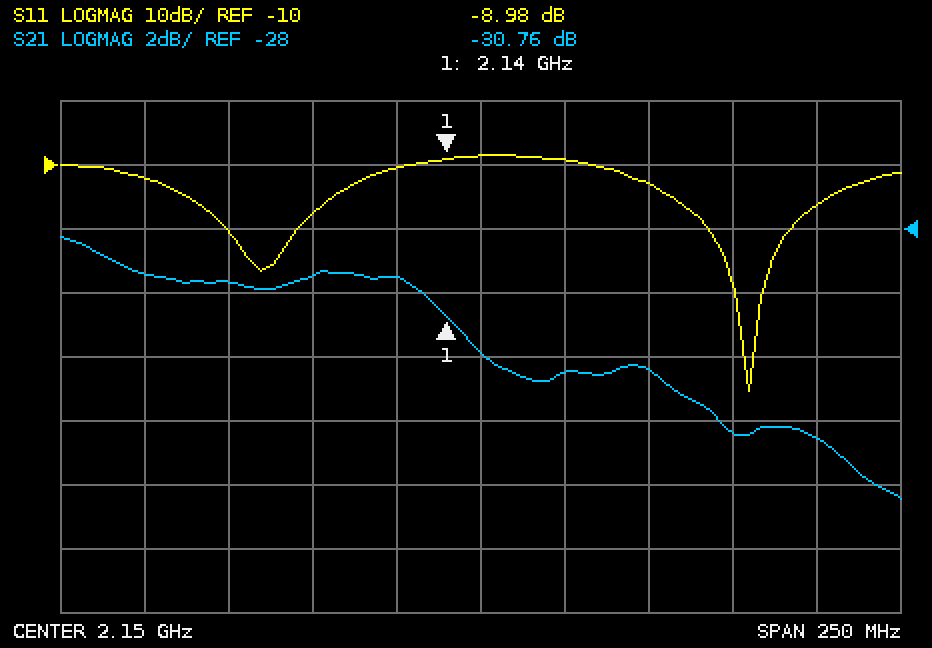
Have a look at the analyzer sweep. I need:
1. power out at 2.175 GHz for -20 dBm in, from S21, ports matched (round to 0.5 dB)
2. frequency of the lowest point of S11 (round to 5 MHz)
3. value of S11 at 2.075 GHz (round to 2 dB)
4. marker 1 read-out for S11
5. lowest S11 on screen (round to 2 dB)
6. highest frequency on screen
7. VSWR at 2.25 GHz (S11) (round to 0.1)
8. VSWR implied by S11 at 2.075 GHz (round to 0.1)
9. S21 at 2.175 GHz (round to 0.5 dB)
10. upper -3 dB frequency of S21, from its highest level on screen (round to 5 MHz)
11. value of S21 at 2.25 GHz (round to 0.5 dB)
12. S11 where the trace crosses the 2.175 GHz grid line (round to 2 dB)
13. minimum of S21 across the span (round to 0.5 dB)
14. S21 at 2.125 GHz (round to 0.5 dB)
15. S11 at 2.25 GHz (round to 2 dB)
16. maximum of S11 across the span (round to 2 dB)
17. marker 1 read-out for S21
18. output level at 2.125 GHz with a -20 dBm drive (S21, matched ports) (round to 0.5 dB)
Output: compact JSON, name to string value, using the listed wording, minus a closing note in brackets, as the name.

{"power out at 2.175 GHz for -20 dBm in, from S21, ports matched": "-52.5 dBm", "frequency of the lowest point of S11": "2.230 GHz", "value of S11 at 2.075 GHz": "-20 dB", "marker 1 read-out for S11": "-8.98 dB", "lowest S11 on screen": "-46 dB", "highest frequency on screen": "2.275 GHz", "VSWR at 2.25 GHz (S11)": "1.4", "VSWR implied by S11 at 2.075 GHz": "1.2", "S21 at 2.175 GHz": "-32.5 dB", "upper -3 dB frequency of S21, from its highest level on screen": "2.145 GHz", "value of S21 at 2.25 GHz": "-34.5 dB", "S11 where the trace crosses the 2.175 GHz grid line": "-10 dB", "minimum of S21 across the span": "-36.5 dB", "S21 at 2.125 GHz": "-29.5 dB", "S11 at 2.25 GHz": "-16 dB", "maximum of S11 across the span": "-8 dB", "marker 1 read-out for S21": "-30.76 dB", "output level at 2.125 GHz with a -20 dBm drive (S21, matched ports)": "-49.5 dBm"}
